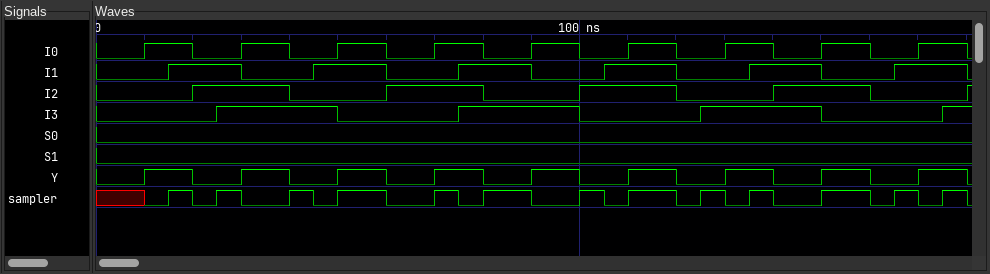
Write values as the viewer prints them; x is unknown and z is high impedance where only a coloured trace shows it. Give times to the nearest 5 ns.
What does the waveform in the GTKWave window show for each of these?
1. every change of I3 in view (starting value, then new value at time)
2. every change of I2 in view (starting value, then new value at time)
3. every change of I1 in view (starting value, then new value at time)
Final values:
0, 1 at 25 ns, 0 at 50 ns, 1 at 75 ns, 0 at 100 ns, 1 at 125 ns, 0 at 150 ns, 1 at 175 ns
0, 1 at 20 ns, 0 at 40 ns, 1 at 60 ns, 0 at 80 ns, 1 at 100 ns, 0 at 120 ns, 1 at 140 ns, 0 at 160 ns, 1 at 180 ns
0, 1 at 15 ns, 0 at 30 ns, 1 at 45 ns, 0 at 60 ns, 1 at 75 ns, 0 at 90 ns, 1 at 105 ns, 0 at 120 ns, 1 at 135 ns, 0 at 150 ns, 1 at 165 ns, 0 at 180 ns
